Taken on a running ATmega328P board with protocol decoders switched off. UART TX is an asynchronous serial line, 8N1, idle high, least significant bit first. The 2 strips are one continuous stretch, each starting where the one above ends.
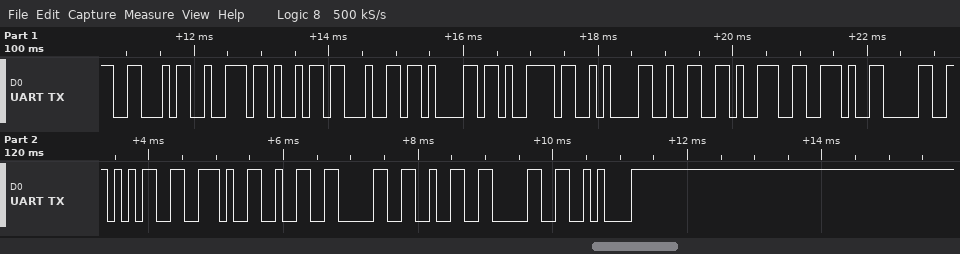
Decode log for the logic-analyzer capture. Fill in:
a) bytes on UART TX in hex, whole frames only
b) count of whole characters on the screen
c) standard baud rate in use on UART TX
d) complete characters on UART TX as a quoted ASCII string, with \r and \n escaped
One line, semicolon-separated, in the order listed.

46 72 69 64 61 79 0A 32 39 2E 30 35 2E 32 30 32 30 0A; 18; 9600 baud; "Friday\n29.05.2020\n"
